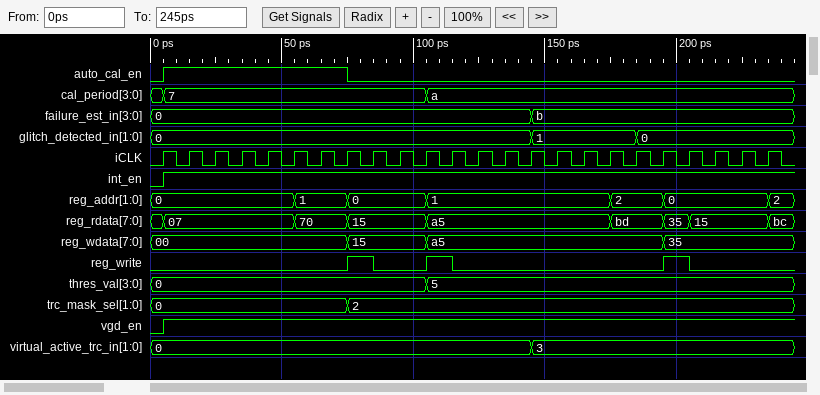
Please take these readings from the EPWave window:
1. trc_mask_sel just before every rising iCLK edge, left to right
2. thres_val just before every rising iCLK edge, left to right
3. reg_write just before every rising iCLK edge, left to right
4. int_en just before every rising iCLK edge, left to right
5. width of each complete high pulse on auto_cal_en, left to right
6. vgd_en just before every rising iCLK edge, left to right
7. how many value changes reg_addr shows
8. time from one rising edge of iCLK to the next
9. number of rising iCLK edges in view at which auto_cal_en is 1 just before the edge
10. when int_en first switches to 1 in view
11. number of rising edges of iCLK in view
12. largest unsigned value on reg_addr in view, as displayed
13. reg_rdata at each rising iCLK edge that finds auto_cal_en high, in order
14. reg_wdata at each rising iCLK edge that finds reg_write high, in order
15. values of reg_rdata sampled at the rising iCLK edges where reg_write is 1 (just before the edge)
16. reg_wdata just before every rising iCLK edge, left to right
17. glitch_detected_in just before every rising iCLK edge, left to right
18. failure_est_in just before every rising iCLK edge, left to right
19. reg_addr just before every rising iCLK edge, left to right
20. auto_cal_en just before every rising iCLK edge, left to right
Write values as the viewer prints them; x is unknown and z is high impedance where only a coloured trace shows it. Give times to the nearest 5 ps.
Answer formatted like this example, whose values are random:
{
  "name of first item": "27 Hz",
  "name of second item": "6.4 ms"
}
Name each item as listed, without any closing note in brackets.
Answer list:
{
  "trc_mask_sel just before every rising iCLK edge, left to right": "0, 0, 0, 0, 0, 0, 0, 0, 2, 2, 2, 2, 2, 2, 2, 2, 2, 2, 2, 2, 2, 2, 2, 2",
  "thres_val just before every rising iCLK edge, left to right": "0, 0, 0, 0, 0, 0, 0, 0, 0, 0, 0, 5, 5, 5, 5, 5, 5, 5, 5, 5, 5, 5, 5, 5",
  "reg_write just before every rising iCLK edge, left to right": "0 0 0 0 0 0 0 0 1 0 0 1 0 0 0 0 0 0 0 0 1 0 0 0",
  "int_en just before every rising iCLK edge, left to right": "0 1 1 1 1 1 1 1 1 1 1 1 1 1 1 1 1 1 1 1 1 1 1 1",
  "width of each complete high pulse on auto_cal_en, left to right": "70 ps",
  "vgd_en just before every rising iCLK edge, left to right": "0 1 1 1 1 1 1 1 1 1 1 1 1 1 1 1 1 1 1 1 1 1 1 1",
  "how many value changes reg_addr shows": "6",
  "time from one rising edge of iCLK to the next": "10 ps",
  "number of rising iCLK edges in view at which auto_cal_en is 1 just before the edge": "7",
  "when int_en first switches to 1 in view": "5 ps",
  "number of rising edges of iCLK in view": "24",
  "largest unsigned value on reg_addr in view, as displayed": "2",
  "reg_rdata at each rising iCLK edge that finds auto_cal_en high, in order": "07, 07, 07, 07, 07, 70, 70",
  "reg_wdata at each rising iCLK edge that finds reg_write high, in order": "15, a5, 35",
  "values of reg_rdata sampled at the rising iCLK edges where reg_write is 1": "15, a5, 35",
  "reg_wdata just before every rising iCLK edge, left to right": "00, 00, 00, 00, 00, 00, 00, 00, 15, 15, 15, a5, a5, a5, a5, a5, a5, a5, a5, a5, 35, 35, 35, 35",
  "glitch_detected_in just before every rising iCLK edge, left to right": "0, 0, 0, 0, 0, 0, 0, 0, 0, 0, 0, 0, 0, 0, 0, 1, 1, 1, 1, 0, 0, 0, 0, 0",
  "failure_est_in just before every rising iCLK edge, left to right": "0, 0, 0, 0, 0, 0, 0, 0, 0, 0, 0, 0, 0, 0, 0, b, b, b, b, b, b, b, b, b",
  "reg_addr just before every rising iCLK edge, left to right": "0, 0, 0, 0, 0, 0, 1, 1, 0, 0, 0, 1, 1, 1, 1, 1, 1, 1, 2, 2, 0, 0, 0, 0",
  "auto_cal_en just before every rising iCLK edge, left to right": "0 1 1 1 1 1 1 1 0 0 0 0 0 0 0 0 0 0 0 0 0 0 0 0"
}
